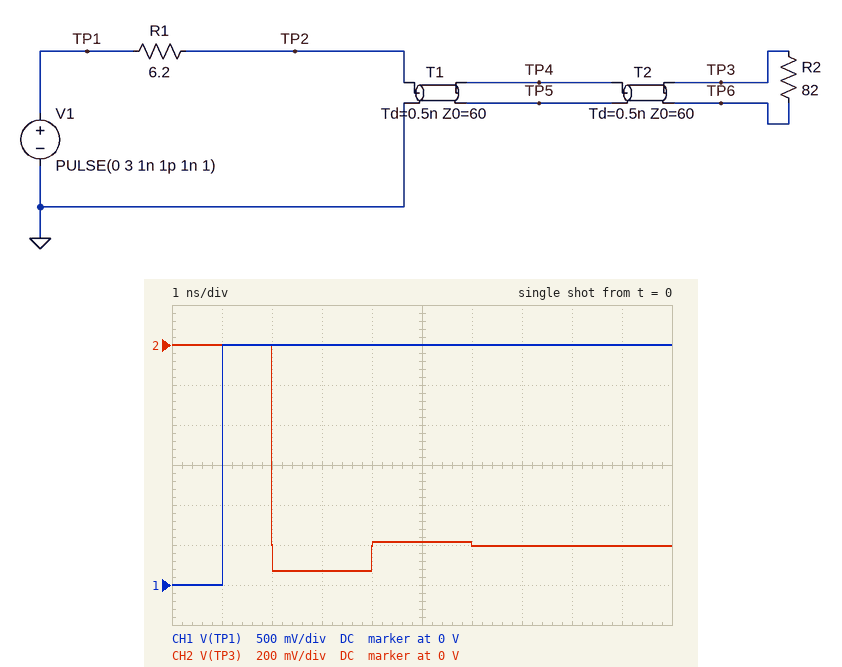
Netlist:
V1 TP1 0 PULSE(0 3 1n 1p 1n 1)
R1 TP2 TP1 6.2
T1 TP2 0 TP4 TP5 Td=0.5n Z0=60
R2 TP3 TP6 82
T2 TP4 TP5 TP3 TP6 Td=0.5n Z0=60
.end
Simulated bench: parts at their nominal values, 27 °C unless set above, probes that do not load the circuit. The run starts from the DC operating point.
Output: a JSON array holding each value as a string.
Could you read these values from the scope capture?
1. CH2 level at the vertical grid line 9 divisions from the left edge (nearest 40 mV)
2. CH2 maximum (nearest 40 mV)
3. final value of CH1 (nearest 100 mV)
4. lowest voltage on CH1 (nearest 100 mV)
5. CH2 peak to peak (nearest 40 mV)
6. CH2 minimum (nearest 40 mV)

["-1.00 V", "0 V", "3.0 V", "0 V", "1.12 V", "-1.12 V"]
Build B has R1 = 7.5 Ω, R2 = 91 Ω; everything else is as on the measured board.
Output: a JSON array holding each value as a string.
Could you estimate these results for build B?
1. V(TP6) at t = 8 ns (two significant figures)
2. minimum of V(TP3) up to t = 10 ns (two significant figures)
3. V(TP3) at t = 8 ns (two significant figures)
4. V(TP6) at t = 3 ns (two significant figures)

["-3.7 V", "-1.0 V", "-900 mV", "-4.3 V"]
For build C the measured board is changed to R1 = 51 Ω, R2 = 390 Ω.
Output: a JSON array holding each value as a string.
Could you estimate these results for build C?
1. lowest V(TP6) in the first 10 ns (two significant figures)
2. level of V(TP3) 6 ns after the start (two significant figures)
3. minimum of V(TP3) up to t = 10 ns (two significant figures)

["-3.0 V", "-200 mV", "-210 mV"]
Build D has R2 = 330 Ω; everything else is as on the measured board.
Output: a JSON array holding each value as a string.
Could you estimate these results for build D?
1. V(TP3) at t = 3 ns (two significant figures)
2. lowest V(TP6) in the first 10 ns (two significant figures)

["-410 mV", "-5.0 V"]
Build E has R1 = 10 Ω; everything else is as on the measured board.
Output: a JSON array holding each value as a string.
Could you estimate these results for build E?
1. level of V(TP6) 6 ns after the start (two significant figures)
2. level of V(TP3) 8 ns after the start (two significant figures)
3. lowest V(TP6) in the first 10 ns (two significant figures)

["-3.6 V", "-960 mV", "-4.0 V"]
